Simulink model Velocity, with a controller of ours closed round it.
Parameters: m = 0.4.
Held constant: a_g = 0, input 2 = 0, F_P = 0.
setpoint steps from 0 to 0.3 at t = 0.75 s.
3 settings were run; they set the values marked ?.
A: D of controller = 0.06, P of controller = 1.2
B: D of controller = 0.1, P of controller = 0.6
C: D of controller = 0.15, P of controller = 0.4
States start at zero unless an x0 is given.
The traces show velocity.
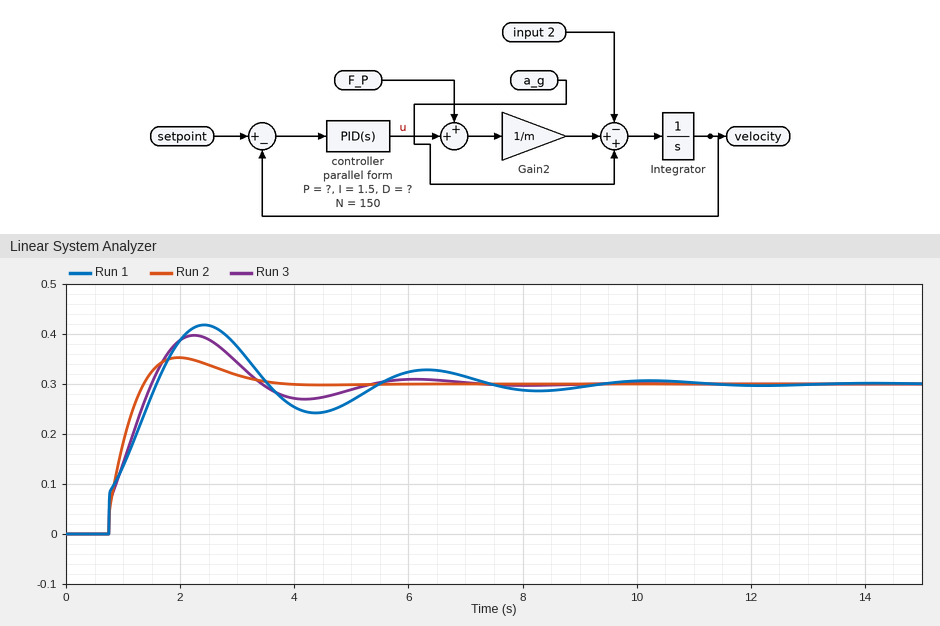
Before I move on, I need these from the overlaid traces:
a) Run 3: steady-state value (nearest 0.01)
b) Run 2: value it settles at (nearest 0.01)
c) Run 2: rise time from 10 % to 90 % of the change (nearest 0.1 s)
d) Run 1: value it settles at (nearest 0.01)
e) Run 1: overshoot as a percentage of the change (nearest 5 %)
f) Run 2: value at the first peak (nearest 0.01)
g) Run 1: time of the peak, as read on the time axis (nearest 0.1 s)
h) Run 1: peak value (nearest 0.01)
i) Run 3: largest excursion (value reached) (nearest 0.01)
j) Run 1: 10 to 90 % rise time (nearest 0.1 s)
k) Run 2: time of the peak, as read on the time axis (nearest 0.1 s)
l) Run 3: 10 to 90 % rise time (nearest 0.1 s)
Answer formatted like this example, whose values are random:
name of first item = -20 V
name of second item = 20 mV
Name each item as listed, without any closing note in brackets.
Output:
Run 3: steady-state value = 0.30
Run 2: value it settles at = 0.30
Run 2: rise time from 10 % to 90 % of the change = 0.5 s
Run 1: value it settles at = 0.30
Run 1: overshoot as a percentage of the change = 40 %
Run 2: value at the first peak = 0.35
Run 1: time of the peak, as read on the time axis = 2.4 s
Run 1: peak value = 0.42
Run 3: largest excursion (value reached) = 0.40
Run 1: 10 to 90 % rise time = 0.7 s
Run 2: time of the peak, as read on the time axis = 2.0 s
Run 3: 10 to 90 % rise time = 0.6 s
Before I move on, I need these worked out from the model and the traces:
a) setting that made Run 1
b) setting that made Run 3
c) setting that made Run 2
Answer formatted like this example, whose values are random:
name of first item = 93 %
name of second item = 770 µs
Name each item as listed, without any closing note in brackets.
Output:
setting that made Run 1 = C
setting that made Run 3 = B
setting that made Run 2 = A
